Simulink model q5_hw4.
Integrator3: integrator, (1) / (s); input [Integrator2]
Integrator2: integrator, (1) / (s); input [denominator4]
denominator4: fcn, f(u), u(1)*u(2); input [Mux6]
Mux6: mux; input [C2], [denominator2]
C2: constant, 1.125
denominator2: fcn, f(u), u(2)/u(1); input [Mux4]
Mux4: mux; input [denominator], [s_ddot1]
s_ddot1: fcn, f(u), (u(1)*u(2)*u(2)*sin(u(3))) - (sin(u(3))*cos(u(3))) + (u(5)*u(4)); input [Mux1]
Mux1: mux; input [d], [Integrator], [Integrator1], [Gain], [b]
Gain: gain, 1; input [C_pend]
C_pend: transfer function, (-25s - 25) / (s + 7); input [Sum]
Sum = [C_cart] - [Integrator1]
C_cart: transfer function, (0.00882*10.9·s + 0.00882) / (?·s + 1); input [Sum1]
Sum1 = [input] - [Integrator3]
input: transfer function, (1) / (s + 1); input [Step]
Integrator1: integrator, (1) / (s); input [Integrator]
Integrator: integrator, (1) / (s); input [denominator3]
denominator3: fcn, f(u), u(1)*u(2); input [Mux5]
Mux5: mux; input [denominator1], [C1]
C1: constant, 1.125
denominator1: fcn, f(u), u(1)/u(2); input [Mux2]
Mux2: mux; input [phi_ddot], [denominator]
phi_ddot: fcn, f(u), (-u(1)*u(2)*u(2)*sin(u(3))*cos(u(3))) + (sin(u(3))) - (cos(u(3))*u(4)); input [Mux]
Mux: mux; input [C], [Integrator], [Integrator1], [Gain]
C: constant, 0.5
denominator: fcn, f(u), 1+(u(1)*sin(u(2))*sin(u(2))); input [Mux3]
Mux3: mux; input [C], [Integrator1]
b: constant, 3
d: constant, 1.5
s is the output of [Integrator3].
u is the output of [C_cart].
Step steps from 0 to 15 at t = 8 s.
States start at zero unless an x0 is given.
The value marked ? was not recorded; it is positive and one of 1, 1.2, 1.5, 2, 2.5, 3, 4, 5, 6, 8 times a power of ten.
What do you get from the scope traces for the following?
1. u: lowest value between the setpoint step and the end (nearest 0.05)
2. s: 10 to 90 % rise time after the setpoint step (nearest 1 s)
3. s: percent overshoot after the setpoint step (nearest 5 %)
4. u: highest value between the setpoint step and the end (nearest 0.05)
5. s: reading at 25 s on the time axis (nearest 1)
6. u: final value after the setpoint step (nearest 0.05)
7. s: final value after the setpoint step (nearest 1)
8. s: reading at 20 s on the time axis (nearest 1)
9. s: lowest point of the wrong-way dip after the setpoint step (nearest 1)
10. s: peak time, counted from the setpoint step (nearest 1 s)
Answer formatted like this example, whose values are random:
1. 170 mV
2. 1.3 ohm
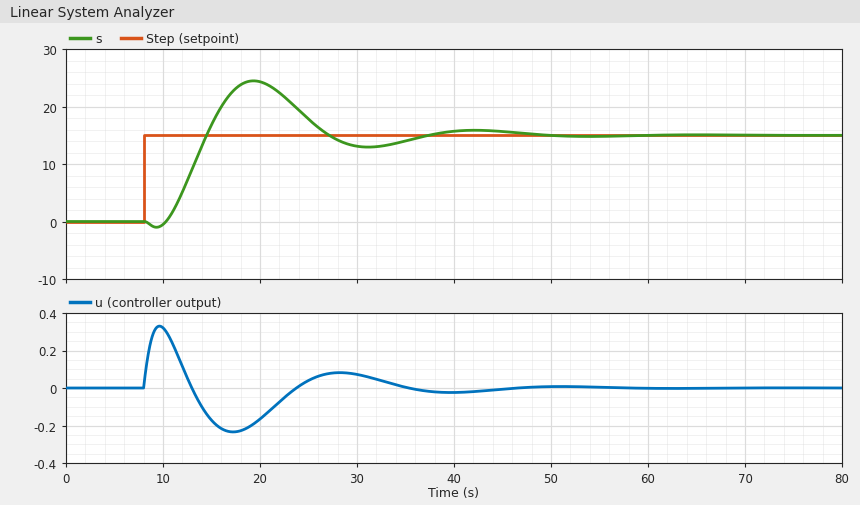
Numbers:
1. -0.25
2. 3 s
3. 65 %
4. 0.35
5. 18
6. 0.00
7. 15
8. 24
9. -1
10. 11 s
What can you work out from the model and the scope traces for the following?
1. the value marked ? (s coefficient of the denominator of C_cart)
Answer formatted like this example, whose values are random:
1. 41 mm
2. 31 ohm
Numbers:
1. 3
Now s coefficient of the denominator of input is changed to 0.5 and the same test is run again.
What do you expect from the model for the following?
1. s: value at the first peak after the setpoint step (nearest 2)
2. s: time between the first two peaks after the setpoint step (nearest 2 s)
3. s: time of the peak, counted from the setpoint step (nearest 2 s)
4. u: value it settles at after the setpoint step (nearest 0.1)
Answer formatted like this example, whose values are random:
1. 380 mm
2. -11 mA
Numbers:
1. 26
2. 22 s
3. 10 s
4. 0.0
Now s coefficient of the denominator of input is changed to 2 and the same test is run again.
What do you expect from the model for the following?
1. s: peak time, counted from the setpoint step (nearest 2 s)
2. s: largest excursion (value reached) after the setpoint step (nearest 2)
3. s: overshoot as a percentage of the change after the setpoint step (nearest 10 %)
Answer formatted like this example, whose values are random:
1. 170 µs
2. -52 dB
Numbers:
1. 12 s
2. 22
3. 50 %
